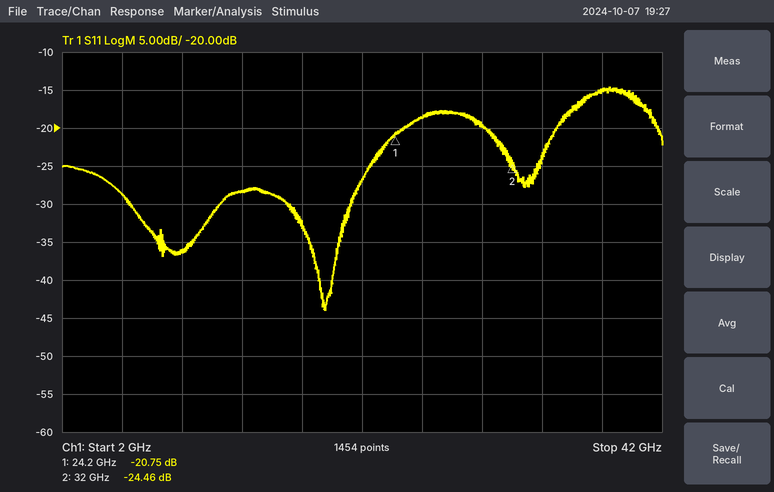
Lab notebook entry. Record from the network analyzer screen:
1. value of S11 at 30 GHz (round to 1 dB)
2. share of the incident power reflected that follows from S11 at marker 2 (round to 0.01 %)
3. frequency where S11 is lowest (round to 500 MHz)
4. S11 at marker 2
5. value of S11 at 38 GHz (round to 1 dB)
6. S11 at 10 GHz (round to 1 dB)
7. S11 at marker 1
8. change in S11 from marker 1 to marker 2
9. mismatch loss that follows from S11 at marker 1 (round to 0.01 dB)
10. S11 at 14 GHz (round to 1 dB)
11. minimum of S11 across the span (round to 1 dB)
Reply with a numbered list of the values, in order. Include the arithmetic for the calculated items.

1. -20 dB
2. 10^(-24.46/10) ≈ 0.36 %
3. 19.5 GHz
4. -24.46 dB
5. -15 dB
6. -36 dB
7. -20.75 dB
8. -24.46 − (-20.75) = -3.71 dB
9. −10 log10(1 − 10^(-20.75/10)) ≈ 0.04 dB
10. -28 dB
11. -44 dB
